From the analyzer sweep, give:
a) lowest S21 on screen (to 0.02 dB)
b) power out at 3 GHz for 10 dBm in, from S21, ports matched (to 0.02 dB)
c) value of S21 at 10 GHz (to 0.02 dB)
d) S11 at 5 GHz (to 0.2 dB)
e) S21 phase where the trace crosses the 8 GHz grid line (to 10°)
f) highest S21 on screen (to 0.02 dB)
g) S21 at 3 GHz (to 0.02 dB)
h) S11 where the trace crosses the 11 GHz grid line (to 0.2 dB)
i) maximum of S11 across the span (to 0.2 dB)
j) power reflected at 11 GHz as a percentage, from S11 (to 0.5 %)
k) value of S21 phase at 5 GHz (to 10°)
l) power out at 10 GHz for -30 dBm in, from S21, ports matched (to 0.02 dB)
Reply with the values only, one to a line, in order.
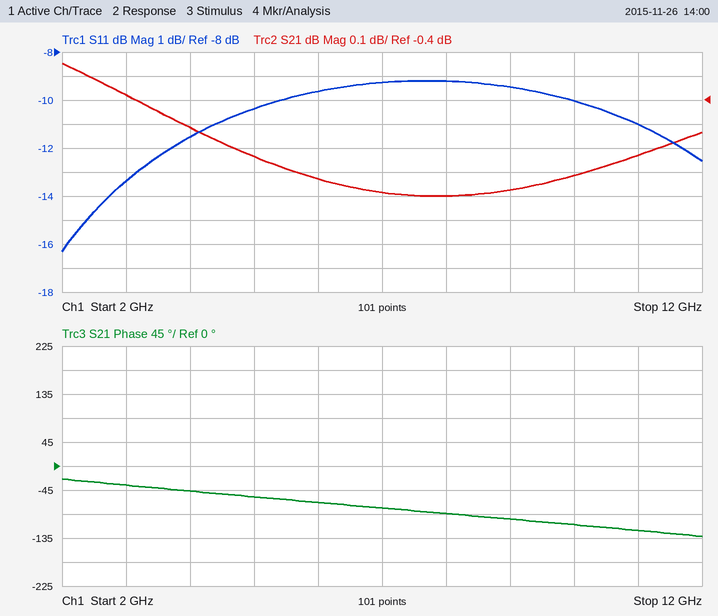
-0.80 dB
9.62 dBm
-0.72 dB
-10.4 dB
-90°
-0.24 dB
-0.38 dB
-11.0 dB
-9.2 dB
8.0 %
-60°
-30.72 dBm
